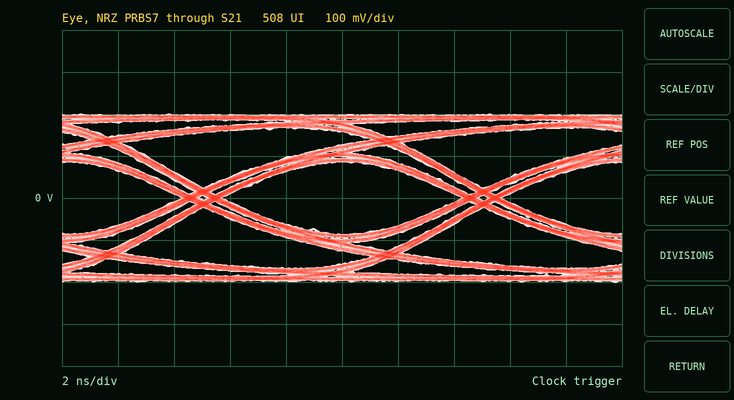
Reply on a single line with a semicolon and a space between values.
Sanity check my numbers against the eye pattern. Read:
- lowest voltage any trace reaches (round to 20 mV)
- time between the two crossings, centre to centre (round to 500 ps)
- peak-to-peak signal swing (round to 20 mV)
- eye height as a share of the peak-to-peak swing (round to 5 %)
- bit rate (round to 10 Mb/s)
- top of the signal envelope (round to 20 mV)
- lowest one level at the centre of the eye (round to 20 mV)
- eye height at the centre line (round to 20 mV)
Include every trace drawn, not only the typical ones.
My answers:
-200 mV; 10.0 ns; 400 mV; 45 %; 100 Mb/s; 200 mV; 80 mV; 180 mV
